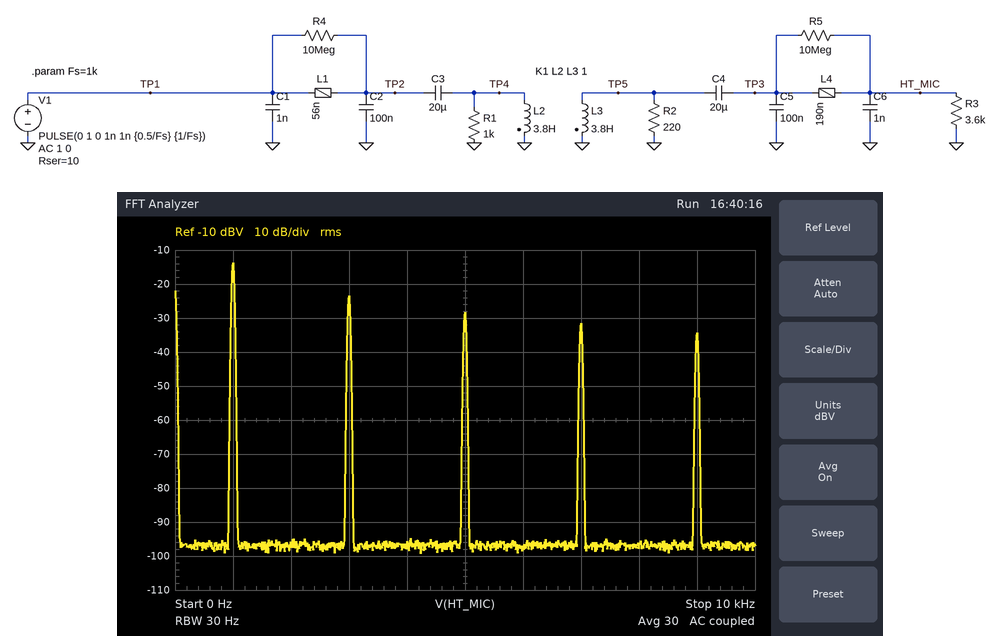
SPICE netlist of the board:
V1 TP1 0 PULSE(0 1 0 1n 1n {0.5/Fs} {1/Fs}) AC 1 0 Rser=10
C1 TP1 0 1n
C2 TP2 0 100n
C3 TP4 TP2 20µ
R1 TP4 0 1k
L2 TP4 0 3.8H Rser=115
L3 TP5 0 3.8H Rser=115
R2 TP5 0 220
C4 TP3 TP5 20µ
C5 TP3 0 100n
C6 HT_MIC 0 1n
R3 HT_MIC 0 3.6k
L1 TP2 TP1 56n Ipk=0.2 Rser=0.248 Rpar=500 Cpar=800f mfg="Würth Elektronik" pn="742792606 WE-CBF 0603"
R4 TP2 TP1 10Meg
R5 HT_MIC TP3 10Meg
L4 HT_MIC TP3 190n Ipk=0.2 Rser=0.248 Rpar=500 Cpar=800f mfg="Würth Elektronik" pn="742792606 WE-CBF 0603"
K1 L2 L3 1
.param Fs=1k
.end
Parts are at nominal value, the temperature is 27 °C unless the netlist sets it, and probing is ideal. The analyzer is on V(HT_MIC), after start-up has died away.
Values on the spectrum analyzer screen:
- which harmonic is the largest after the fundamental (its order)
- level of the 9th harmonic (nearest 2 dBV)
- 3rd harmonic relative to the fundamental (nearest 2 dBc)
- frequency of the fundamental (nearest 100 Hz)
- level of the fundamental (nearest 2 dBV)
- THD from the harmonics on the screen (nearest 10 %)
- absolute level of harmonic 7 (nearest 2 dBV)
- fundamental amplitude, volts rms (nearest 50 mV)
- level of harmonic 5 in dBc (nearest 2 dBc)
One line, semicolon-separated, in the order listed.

3; -34 dBV; -10 dBc; 1.0 kHz; -14 dBV; 40 %; -32 dBV; 200 mV; -14 dBc
